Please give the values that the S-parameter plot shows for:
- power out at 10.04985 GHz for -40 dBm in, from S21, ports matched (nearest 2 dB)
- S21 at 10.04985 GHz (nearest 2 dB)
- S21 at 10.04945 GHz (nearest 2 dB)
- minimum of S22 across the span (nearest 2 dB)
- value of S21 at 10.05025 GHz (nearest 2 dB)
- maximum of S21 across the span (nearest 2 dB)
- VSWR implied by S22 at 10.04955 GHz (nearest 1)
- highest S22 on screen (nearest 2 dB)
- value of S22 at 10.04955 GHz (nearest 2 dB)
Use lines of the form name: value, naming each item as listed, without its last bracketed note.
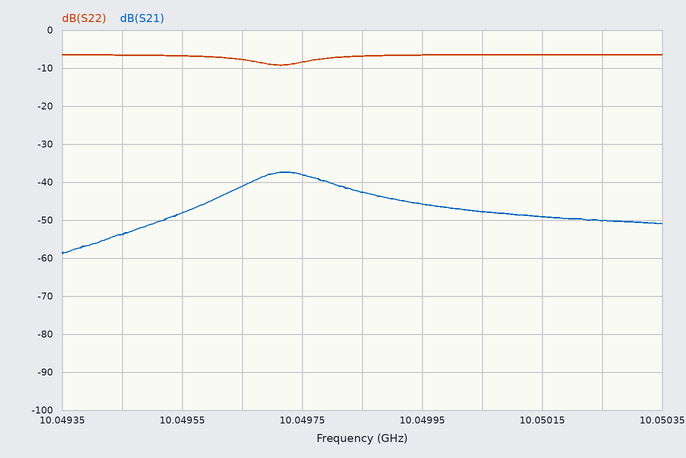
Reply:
power out at 10.04985 GHz for -40 dBm in, from S21, ports matched: -82 dBm
S21 at 10.04985 GHz: -42 dB
S21 at 10.04945 GHz: -54 dB
minimum of S22 across the span: -10 dB
value of S21 at 10.05025 GHz: -50 dB
maximum of S21 across the span: -38 dB
VSWR implied by S22 at 10.04955 GHz: 3
highest S22 on screen: -6 dB
value of S22 at 10.04955 GHz: -6 dB
